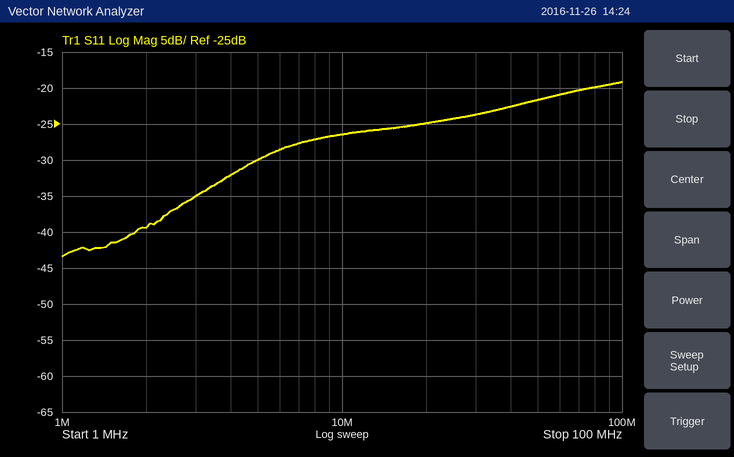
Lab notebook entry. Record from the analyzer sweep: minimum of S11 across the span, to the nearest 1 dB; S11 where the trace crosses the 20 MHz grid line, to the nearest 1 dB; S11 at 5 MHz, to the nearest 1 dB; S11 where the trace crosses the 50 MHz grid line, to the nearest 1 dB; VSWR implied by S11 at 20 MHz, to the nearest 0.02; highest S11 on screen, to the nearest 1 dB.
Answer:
-43 dB
-25 dB
-30 dB
-22 dB
1.12
-19 dB
